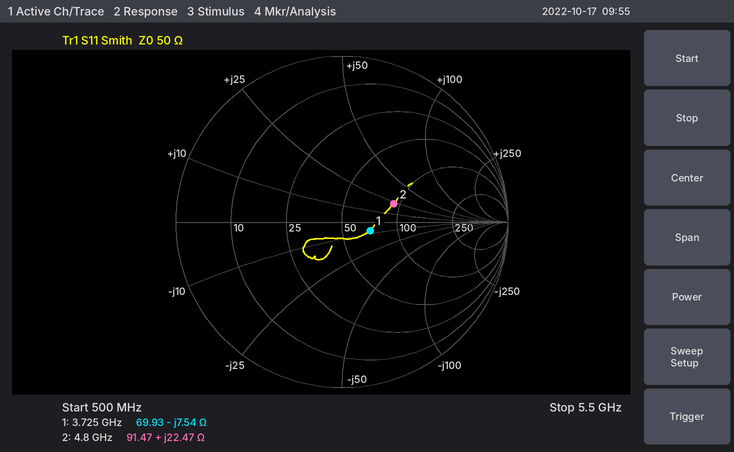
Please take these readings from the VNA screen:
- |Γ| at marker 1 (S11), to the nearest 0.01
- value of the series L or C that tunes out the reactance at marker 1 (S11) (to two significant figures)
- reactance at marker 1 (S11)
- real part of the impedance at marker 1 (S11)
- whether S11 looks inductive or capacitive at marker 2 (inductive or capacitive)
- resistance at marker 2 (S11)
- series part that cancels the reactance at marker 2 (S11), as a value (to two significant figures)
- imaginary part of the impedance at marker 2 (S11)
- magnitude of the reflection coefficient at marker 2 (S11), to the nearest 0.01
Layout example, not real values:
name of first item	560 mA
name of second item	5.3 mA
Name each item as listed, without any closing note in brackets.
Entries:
|Γ| at marker 1 (S11), to the nearest 0.01	0.18
value of the series L or C that tunes out the reactance at marker 1 (S11)	320 pH
reactance at marker 1	-7.54 Ω
real part of the impedance at marker 1	69.93 Ω
whether S11 looks inductive or capacitive at marker 2	inductive
resistance at marker 2	91.47 Ω
series part that cancels the reactance at marker 2 (S11), as a value	1.5 pF
imaginary part of the impedance at marker 2	+22.47 Ω
magnitude of the reflection coefficient at marker 2 (S11), to the nearest 0.01	0.33
